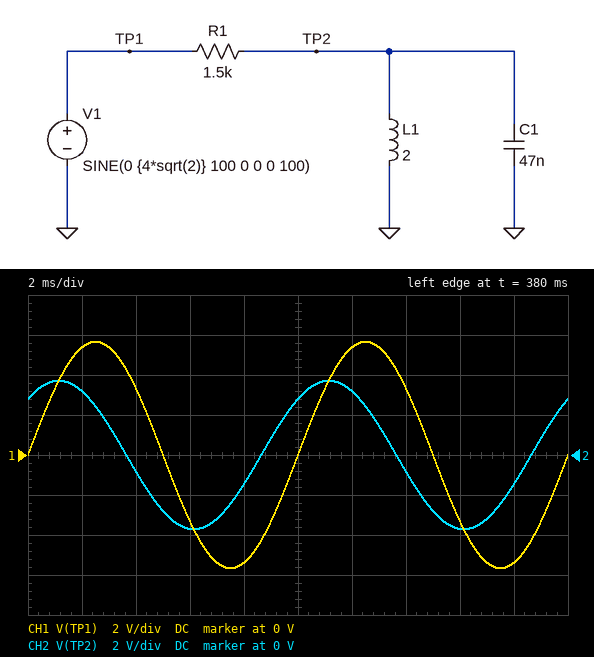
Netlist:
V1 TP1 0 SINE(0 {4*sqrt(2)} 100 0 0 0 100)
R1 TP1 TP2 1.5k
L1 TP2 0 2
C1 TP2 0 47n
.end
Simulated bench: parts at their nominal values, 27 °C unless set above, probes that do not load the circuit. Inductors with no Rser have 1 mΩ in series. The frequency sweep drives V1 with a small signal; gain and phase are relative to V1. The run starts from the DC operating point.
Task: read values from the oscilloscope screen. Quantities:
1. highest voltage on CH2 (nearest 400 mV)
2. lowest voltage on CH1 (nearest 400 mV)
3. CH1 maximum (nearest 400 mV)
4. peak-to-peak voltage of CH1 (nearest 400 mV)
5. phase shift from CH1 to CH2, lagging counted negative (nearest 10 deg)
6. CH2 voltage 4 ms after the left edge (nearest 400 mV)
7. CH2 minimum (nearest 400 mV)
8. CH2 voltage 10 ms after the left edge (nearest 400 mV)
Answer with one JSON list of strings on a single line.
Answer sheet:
["3.6 V", "-5.6 V", "5.6 V", "11.2 V", "50 deg", "-800 mV", "-3.6 V", "2.8 V"]
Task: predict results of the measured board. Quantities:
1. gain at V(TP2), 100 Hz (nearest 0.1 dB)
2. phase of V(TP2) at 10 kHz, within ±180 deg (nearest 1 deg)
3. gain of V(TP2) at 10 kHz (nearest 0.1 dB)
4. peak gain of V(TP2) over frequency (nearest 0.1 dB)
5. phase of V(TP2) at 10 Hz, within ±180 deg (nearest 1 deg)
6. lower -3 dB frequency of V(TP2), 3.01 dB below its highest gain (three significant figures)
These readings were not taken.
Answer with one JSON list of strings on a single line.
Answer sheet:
["-3.7 dB", "-77 deg", "-13.1 dB", "0 dB", "85 deg", "114 Hz"]
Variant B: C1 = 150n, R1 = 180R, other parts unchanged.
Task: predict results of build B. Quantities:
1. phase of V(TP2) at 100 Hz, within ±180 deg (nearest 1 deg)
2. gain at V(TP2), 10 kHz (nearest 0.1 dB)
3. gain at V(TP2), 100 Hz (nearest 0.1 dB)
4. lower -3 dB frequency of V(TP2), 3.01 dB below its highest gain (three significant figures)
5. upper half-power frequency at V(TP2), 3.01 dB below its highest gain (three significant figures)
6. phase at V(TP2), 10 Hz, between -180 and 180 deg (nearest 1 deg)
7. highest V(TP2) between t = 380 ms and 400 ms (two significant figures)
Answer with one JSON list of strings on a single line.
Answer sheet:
["7 deg", "-5.9 dB", "-0.1 dB", "14.3 Hz", "5.91 kHz", "55 deg", "5.6 V"]
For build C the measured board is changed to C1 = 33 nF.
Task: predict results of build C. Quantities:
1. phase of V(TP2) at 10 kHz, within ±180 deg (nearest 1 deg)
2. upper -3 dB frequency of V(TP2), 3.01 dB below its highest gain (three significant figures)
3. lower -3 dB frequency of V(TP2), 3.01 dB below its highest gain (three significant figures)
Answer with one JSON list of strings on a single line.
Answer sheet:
["-72 deg", "3.33 kHz", "115 Hz"]
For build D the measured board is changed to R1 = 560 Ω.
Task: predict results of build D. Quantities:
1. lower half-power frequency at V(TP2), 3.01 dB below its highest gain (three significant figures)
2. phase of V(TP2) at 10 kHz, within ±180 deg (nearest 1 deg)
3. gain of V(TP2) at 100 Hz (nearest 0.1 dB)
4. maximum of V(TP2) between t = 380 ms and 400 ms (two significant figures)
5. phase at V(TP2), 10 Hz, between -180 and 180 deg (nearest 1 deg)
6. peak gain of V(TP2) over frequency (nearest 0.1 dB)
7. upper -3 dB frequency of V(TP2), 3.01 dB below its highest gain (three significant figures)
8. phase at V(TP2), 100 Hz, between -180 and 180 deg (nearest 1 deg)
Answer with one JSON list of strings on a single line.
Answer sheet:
["44.2 Hz", "-59 deg", "-0.7 dB", "5.2 V", "77 deg", "0 dB", "6.09 kHz", "23 deg"]
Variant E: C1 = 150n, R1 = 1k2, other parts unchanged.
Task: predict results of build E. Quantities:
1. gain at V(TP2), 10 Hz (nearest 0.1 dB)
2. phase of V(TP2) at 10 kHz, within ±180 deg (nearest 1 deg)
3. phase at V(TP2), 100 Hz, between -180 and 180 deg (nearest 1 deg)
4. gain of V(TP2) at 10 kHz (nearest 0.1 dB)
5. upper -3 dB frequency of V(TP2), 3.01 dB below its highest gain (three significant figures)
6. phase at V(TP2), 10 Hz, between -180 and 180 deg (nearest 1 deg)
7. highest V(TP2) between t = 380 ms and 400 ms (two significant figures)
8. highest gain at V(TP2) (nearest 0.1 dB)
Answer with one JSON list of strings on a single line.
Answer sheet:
["-19.6 dB", "-85 deg", "40 deg", "-21.1 dB", "971 Hz", "84 deg", "4.3 V", "0 dB"]
